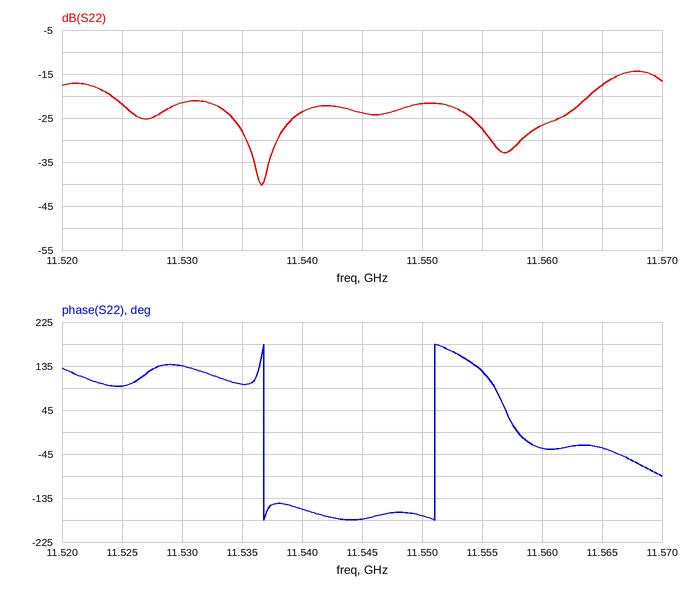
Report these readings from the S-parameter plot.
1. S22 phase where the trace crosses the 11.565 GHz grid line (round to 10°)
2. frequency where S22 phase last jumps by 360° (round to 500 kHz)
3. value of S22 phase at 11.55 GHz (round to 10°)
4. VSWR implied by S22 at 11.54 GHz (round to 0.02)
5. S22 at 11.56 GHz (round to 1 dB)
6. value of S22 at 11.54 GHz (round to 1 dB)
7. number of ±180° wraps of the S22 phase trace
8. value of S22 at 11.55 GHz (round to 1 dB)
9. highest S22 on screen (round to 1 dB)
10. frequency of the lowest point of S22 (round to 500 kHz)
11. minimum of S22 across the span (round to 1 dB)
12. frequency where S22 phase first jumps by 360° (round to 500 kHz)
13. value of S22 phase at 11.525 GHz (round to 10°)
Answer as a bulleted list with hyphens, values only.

- -30°
- 11.5510 GHz
- -170°
- 1.14
- -27 dB
- -24 dB
- 2
- -22 dB
- -14 dB
- 11.5365 GHz
- -40 dB
- 11.5370 GHz
- 90°
